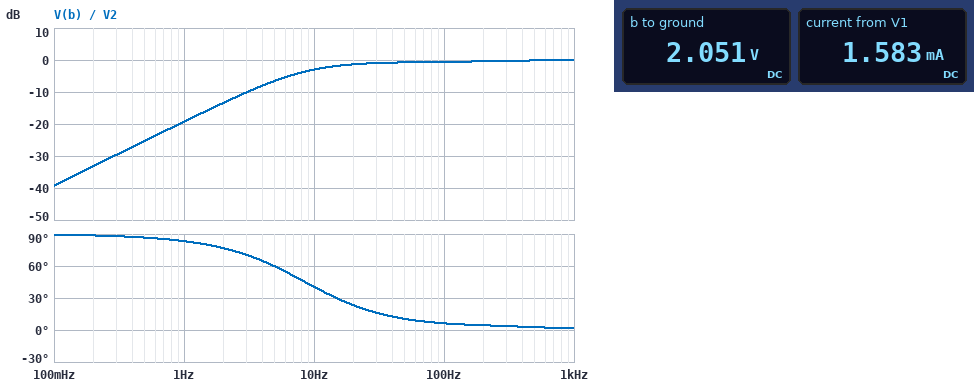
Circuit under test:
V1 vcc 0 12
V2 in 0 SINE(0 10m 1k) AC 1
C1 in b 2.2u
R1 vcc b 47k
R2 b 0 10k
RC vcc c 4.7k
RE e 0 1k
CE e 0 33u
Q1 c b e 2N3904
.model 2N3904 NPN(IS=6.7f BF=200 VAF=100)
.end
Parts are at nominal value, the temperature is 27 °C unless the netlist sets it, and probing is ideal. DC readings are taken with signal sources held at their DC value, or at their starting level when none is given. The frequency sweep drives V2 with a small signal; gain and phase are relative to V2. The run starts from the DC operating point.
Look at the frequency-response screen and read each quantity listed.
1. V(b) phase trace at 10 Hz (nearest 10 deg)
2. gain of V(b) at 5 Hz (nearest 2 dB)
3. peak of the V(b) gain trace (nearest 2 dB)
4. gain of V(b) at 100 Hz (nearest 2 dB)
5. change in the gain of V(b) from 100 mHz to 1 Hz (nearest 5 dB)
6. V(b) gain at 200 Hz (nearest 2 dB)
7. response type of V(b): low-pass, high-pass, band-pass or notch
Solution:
40 deg
-6 dB
0 dB
0 dB
20 dB
0 dB
high-pass
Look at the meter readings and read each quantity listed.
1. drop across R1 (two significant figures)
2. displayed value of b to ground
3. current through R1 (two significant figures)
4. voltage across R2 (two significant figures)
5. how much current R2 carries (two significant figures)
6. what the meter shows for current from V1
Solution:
9.9 V
2.051 V
210 µA
2.1 V
210 µA
1.583 mA
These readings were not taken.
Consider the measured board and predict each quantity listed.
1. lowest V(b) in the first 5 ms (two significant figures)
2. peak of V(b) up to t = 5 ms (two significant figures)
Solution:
2.0 V
2.1 V
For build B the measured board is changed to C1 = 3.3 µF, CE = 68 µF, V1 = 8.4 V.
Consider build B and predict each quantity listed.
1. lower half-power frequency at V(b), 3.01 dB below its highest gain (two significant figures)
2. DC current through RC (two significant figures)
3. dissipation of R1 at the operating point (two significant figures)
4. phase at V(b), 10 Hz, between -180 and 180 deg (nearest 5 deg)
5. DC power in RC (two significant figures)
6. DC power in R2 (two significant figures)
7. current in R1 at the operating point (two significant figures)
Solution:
6.9 Hz
780 µA
1.0 mW
30 deg
2.9 mW
210 µW
150 µA
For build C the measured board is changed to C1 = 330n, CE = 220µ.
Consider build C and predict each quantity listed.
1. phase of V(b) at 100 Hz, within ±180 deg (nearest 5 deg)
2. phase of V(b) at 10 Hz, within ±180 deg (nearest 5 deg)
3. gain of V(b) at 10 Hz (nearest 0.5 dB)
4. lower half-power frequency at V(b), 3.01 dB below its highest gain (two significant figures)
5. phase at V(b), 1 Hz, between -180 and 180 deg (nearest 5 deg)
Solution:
50 deg
60 deg
-18.0 dB
200 Hz
85 deg
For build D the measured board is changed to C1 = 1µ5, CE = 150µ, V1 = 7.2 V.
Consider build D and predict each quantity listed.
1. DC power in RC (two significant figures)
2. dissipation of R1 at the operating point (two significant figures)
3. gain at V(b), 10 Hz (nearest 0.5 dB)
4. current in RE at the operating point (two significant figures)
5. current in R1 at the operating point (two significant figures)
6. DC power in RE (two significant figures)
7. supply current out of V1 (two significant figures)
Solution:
1.6 mW
760 µW
-6.0 dB
590 µA
130 µA
350 µW
710 µA
